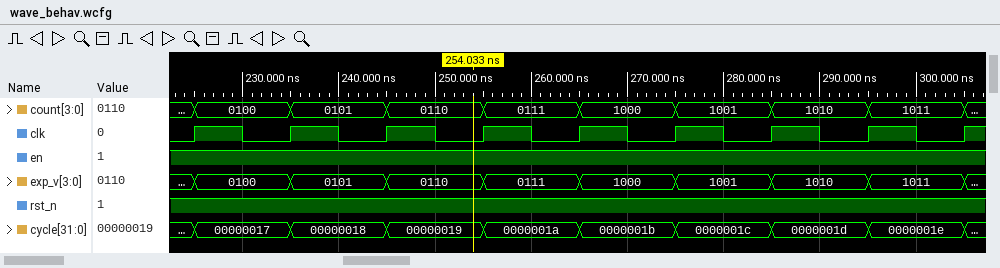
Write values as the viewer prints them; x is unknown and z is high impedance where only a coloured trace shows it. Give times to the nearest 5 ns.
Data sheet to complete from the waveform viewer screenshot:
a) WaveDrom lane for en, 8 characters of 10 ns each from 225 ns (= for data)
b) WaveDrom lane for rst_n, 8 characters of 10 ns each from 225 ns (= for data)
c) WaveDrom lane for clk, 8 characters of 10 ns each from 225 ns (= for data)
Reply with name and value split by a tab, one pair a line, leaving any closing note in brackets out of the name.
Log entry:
WaveDrom lane for en, 8 characters of 10 ns each from 225 ns	{name: 'en', wave: '1.......'}
WaveDrom lane for rst_n, 8 characters of 10 ns each from 225 ns	{name: 'rst_n', wave: '1.......'}
WaveDrom lane for clk, 8 characters of 10 ns each from 225 ns	{name: 'clk', wave: 'p.......'}
